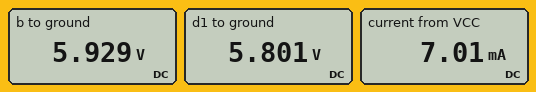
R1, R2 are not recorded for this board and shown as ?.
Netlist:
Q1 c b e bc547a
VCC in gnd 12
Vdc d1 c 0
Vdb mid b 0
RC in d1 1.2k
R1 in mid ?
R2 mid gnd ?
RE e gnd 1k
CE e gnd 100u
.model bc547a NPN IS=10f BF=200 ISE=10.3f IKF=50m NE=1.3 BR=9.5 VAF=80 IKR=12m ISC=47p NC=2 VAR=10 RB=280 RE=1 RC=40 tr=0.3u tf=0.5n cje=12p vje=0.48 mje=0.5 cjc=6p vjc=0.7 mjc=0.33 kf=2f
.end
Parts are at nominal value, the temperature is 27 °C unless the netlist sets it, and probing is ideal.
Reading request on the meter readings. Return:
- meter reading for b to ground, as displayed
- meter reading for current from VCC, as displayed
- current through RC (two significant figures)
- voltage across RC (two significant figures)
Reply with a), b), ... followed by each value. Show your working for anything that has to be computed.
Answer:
a) 5.929 V
b) 7.01 mA
c) (12 V - 5.801 V) / 1.2 kΩ = 5.2 mA
d) 12 V - 5.801 V = 6.2 V
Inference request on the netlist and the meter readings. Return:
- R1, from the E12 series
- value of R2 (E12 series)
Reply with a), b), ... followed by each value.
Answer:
a) 3.3 kΩ
b) 3.3 kΩ
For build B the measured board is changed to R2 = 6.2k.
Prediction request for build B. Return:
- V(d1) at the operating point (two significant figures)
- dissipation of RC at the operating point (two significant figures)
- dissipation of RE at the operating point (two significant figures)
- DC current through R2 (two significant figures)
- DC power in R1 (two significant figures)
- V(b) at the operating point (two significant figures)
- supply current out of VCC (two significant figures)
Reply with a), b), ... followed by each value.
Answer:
a) 5.9 V
b) 31 mW
c) 32 mW
d) 1.1 mA
e) 9.0 mW
f) 6.6 V
g) 6.7 mA
